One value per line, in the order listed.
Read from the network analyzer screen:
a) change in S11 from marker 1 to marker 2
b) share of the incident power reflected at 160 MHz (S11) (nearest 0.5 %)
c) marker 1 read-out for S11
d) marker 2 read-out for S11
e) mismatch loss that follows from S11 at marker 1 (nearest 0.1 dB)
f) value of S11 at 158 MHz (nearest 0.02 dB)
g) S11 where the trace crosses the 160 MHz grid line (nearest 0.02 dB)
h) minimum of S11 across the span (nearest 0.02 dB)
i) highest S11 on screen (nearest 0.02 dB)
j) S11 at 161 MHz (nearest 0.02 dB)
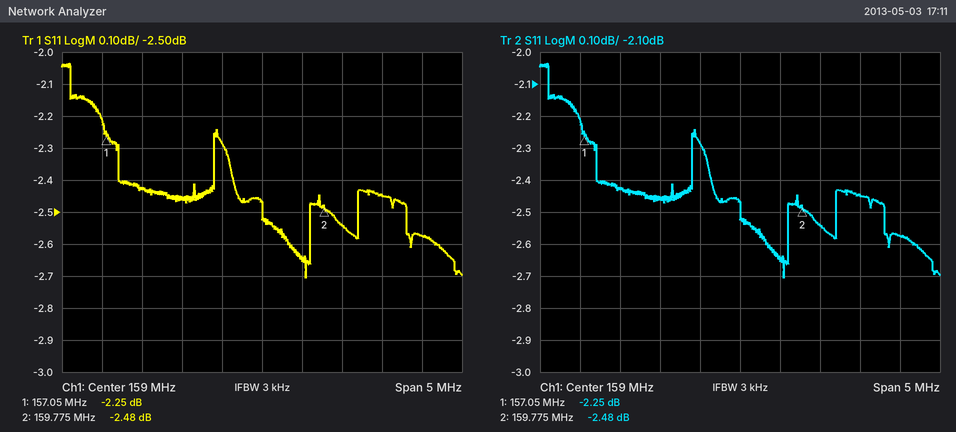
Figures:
-0.23 dB
55.5 %
-2.25 dB
-2.48 dB
3.9 dB
-2.46 dB
-2.54 dB
-2.70 dB
-2.04 dB
-2.58 dB
